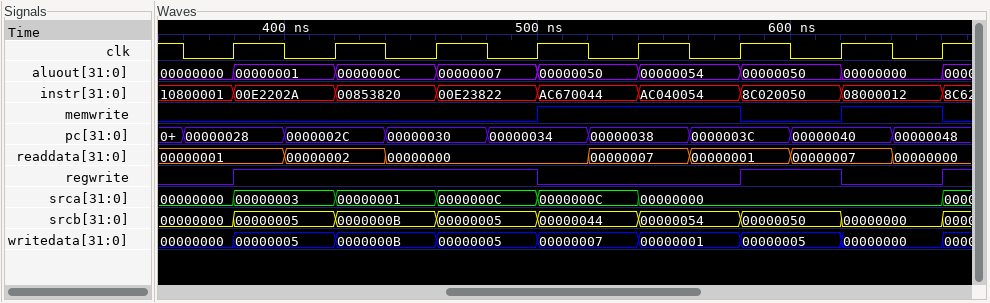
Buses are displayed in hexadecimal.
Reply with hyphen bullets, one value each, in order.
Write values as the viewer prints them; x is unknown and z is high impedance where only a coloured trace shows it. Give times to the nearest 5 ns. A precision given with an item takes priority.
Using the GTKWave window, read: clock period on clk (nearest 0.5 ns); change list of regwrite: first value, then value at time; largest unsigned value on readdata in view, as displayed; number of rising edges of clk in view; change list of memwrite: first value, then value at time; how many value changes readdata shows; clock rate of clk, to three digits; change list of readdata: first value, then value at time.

- 40 ns
- 0, 1 at 380 ns, 0 at 500 ns, 1 at 580 ns, 0 at 620 ns, 1 at 660 ns
- 00000007
- 8
- 0, 1 at 500 ns, 0 at 580 ns, 1 at 620 ns, 0 at 660 ns
- 6
- 25.0 MHz
- 00000001, 00000002 at 400 ns, 00000000 at 440 ns, 00000007 at 520 ns, 00000001 at 560 ns, 00000007 at 600 ns, 00000000 at 640 ns
